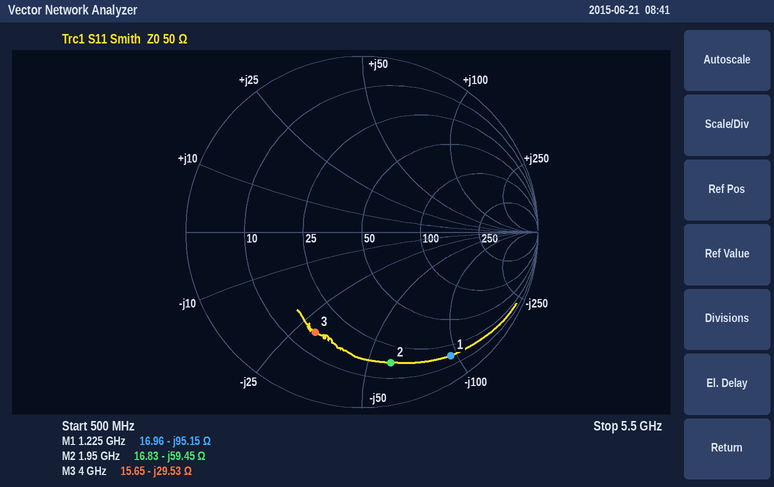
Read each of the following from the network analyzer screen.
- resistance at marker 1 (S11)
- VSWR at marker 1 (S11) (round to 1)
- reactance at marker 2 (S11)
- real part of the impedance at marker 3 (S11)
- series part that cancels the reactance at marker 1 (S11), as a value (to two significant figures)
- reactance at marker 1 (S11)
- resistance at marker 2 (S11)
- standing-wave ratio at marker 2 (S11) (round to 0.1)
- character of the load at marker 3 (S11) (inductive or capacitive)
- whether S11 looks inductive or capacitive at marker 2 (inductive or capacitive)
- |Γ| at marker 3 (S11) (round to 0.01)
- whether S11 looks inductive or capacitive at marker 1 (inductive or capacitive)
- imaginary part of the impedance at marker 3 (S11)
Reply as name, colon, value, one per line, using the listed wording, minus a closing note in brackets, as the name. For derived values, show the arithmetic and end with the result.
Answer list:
resistance at marker 1: 16.96 Ω
VSWR at marker 1 (S11): 14
reactance at marker 2: -59.45 Ω
real part of the impedance at marker 3: 15.65 Ω
series part that cancels the reactance at marker 1 (S11), as a value: L = 95.15 Ω/(2π × 1.225 GHz) ≈ 12 nH
reactance at marker 1: -95.15 Ω
resistance at marker 2: 16.83 Ω
standing-wave ratio at marker 2 (S11): 7.4
character of the load at marker 3 (S11): capacitive
whether S11 looks inductive or capacitive at marker 2: capacitive
|Γ| at marker 3 (S11): 0.63
whether S11 looks inductive or capacitive at marker 1: capacitive
imaginary part of the impedance at marker 3: -29.53 Ω
